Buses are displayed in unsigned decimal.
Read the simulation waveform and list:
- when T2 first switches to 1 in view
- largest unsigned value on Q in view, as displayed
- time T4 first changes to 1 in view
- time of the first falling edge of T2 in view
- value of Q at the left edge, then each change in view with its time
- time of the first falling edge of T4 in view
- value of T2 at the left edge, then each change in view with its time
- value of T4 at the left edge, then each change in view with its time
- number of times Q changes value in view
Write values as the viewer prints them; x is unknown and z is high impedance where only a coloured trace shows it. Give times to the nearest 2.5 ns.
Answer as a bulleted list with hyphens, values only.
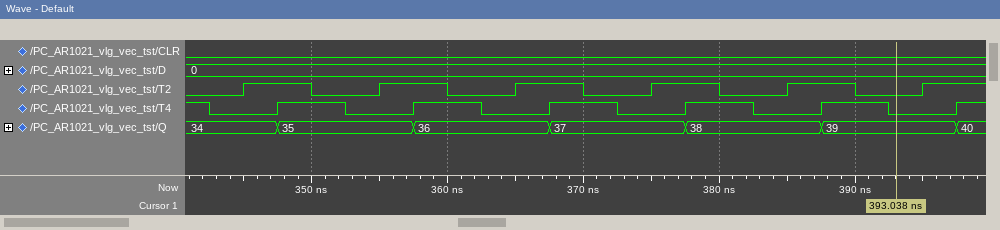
- 345 ns
- 40
- 347.5 ns
- 350 ns
- 34, 35 at 347.5 ns, 36 at 357.5 ns, 37 at 367.5 ns, 38 at 377.5 ns, 39 at 387.5 ns, 40 at 397.5 ns
- 342.5 ns
- 0, 1 at 345 ns, 0 at 350 ns, 1 at 355 ns, 0 at 360 ns, 1 at 365 ns, 0 at 370 ns, 1 at 375 ns, 0 at 380 ns, 1 at 385 ns, 0 at 390 ns, 1 at 395 ns
- 1, 0 at 342.5 ns, 1 at 347.5 ns, 0 at 352.5 ns, 1 at 357.5 ns, 0 at 362.5 ns, 1 at 367.5 ns, 0 at 372.5 ns, 1 at 377.5 ns, 0 at 382.5 ns, 1 at 387.5 ns, 0 at 392.5 ns, 1 at 397.5 ns
- 6
